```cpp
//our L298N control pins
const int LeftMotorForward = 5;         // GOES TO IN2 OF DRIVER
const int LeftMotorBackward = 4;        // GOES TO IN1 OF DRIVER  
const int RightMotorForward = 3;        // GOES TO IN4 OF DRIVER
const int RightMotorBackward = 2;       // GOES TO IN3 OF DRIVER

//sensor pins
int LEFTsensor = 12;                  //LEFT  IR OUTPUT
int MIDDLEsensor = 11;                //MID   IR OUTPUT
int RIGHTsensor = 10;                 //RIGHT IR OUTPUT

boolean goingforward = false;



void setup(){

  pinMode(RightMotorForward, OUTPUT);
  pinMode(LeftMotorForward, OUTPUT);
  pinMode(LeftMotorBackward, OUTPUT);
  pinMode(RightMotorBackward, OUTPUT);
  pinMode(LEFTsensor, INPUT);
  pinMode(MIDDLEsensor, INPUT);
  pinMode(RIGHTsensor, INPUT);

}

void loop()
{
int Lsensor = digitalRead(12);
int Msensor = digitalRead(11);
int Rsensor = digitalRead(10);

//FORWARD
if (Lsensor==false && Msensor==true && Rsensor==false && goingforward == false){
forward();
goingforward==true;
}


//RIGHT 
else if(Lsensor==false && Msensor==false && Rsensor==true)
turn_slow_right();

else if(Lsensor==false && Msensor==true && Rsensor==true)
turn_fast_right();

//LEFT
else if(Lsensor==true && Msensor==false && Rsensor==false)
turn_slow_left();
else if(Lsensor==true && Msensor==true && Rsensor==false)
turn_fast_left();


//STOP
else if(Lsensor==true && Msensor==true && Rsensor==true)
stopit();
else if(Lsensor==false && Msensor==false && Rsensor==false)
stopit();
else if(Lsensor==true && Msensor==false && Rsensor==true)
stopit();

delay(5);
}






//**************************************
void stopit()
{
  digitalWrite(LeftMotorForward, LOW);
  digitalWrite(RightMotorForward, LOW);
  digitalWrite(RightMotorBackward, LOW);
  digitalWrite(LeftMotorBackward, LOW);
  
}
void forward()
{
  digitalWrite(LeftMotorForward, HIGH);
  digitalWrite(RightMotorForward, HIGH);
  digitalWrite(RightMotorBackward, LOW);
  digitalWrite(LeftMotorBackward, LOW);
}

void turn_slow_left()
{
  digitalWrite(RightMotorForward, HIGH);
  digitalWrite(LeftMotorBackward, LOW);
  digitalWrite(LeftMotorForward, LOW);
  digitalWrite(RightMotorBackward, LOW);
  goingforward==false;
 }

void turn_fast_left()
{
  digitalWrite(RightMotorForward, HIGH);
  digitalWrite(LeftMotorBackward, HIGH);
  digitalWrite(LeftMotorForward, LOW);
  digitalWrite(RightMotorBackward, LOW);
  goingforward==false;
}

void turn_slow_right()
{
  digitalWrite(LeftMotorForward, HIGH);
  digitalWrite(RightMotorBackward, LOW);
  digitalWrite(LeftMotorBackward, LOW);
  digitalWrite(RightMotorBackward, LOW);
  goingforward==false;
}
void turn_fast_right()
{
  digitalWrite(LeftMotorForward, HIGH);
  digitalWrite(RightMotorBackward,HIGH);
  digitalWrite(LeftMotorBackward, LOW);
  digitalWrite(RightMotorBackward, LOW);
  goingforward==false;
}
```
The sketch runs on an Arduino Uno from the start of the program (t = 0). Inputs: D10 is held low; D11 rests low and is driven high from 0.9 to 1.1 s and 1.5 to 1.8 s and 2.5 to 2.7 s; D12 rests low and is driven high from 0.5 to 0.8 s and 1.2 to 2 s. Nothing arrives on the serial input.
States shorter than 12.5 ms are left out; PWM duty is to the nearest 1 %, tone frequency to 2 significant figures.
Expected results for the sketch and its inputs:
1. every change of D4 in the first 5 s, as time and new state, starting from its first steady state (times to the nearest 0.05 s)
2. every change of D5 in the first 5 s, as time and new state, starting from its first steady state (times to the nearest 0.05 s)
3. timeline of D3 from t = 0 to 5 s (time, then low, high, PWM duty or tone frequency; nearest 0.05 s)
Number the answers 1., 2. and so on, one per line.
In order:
1. 0 s low; 1.5 s high; 1.8 s low
2. 0 s low; 0.9 s high; 1.1 s low; 2.5 s high; 2.7 s low
3. 0 s low; 0.5 s high; 0.8 s low; 0.9 s high; 1.1 s low; 1.2 s high; 2 s low; 2.5 s high; 2.7 s low
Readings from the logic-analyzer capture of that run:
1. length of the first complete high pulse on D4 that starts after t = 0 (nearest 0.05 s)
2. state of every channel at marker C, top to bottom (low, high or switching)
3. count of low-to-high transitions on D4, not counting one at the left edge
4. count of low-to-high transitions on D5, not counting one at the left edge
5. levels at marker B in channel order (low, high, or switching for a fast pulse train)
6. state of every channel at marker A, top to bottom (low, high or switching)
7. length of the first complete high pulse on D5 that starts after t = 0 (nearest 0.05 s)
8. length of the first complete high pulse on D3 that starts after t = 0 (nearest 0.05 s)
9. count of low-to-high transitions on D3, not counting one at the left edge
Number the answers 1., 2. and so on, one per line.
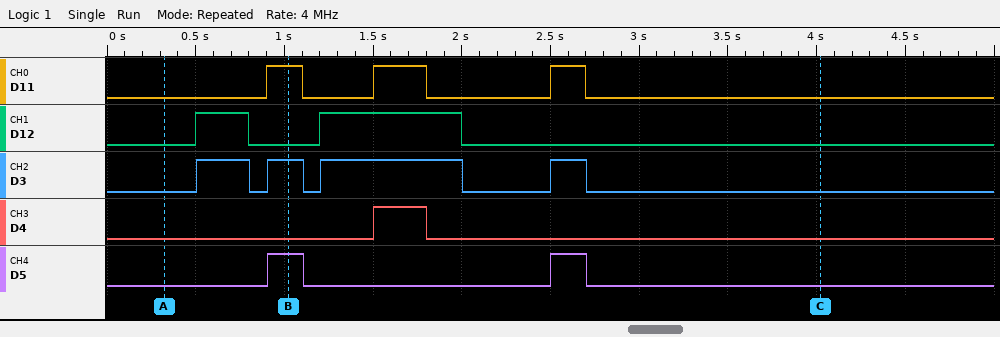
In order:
1. 0.30 s
2. D11 low, D12 low, D3 low, D4 low, D5 low
3. 1
4. 2
5. D11 high, D12 low, D3 high, D4 low, D5 high
6. D11 low, D12 low, D3 low, D4 low, D5 low
7. 0.20 s
8. 0.30 s
9. 4
